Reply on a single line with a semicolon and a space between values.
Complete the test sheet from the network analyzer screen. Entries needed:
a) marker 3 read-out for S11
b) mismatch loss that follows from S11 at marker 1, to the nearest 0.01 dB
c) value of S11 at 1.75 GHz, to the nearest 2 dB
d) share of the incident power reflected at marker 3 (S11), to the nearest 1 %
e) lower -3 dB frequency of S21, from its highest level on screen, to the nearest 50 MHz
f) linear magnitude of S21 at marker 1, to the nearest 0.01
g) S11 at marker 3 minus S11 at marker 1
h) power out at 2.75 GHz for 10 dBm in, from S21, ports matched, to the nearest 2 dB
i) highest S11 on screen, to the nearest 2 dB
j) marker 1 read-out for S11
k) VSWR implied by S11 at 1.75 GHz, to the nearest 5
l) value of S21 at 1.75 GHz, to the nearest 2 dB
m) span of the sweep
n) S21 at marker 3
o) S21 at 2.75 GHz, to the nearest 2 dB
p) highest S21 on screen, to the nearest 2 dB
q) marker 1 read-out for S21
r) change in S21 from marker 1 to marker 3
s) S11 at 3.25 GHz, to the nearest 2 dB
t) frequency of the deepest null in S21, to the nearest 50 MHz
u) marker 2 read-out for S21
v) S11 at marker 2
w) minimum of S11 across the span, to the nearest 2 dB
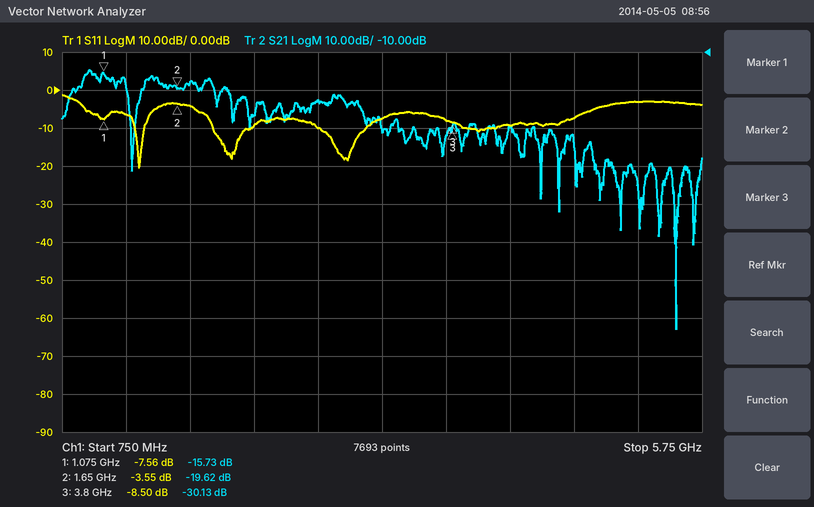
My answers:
-8.50 dB; 0.84 dB; -4 dB; 14 %; 900 MHz; 0.16; -0.94 dB; -12 dBm; -2 dB; -7.56 dB; 5; -18 dB; 5 GHz; -30.13 dB; -22 dB; -14 dB; -15.73 dB; -14.40 dB; -8 dB; 5.55 GHz; -19.62 dB; -3.55 dB; -20 dB
